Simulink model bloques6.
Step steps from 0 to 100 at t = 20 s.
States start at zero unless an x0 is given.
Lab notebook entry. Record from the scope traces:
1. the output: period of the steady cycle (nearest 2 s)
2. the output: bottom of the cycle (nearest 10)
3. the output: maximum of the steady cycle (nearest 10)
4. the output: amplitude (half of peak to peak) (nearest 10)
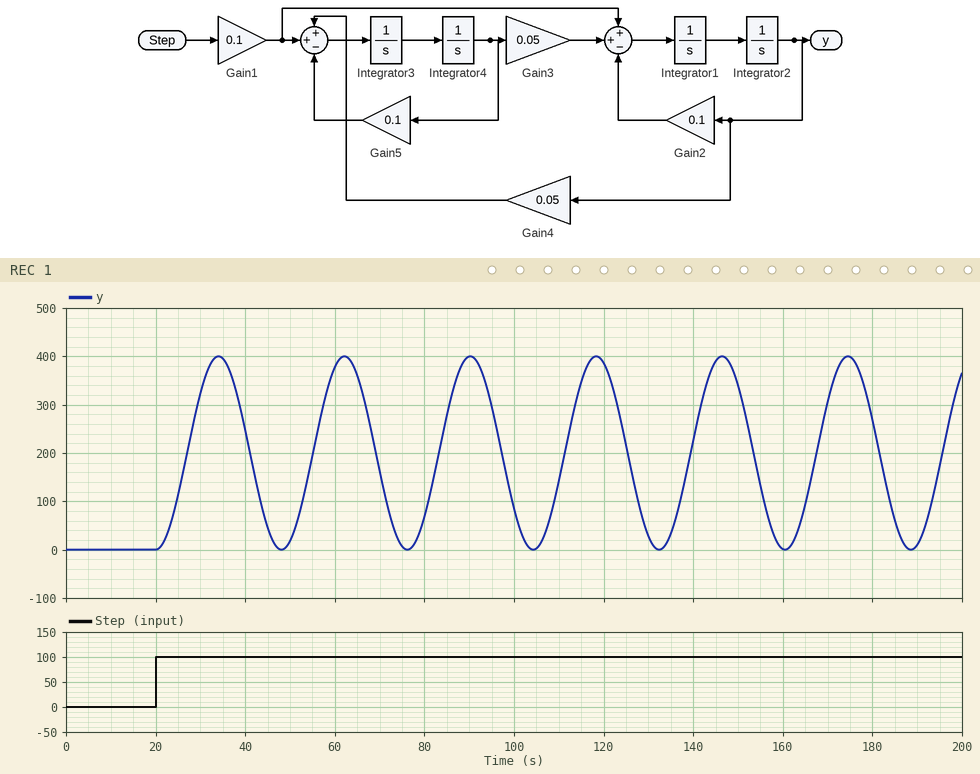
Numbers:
28 s
0
400
200
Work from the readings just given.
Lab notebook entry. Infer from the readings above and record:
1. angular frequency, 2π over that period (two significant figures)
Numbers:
0.22 rad/s
